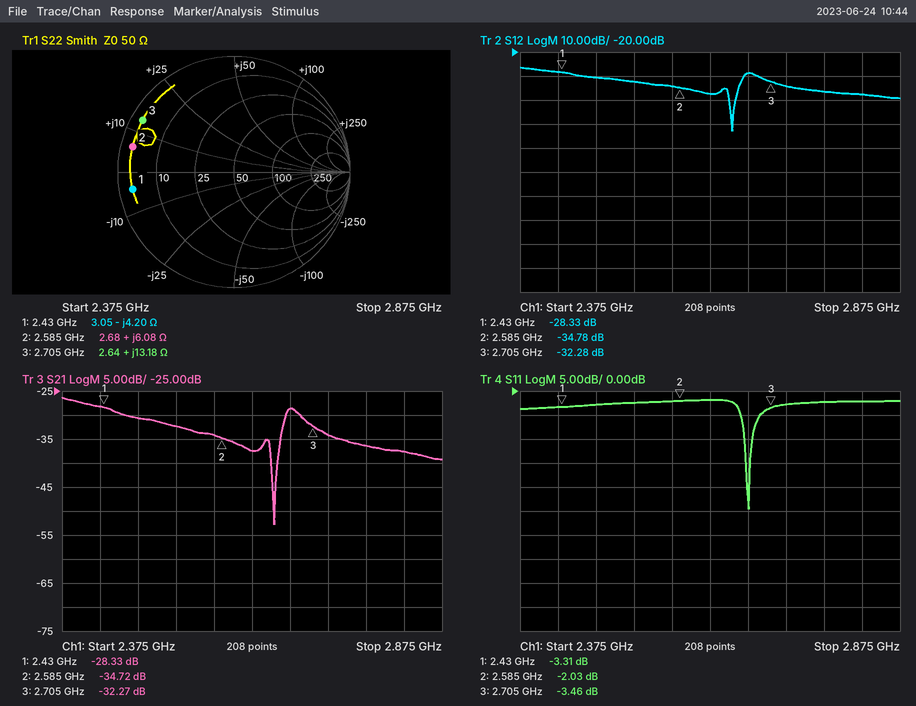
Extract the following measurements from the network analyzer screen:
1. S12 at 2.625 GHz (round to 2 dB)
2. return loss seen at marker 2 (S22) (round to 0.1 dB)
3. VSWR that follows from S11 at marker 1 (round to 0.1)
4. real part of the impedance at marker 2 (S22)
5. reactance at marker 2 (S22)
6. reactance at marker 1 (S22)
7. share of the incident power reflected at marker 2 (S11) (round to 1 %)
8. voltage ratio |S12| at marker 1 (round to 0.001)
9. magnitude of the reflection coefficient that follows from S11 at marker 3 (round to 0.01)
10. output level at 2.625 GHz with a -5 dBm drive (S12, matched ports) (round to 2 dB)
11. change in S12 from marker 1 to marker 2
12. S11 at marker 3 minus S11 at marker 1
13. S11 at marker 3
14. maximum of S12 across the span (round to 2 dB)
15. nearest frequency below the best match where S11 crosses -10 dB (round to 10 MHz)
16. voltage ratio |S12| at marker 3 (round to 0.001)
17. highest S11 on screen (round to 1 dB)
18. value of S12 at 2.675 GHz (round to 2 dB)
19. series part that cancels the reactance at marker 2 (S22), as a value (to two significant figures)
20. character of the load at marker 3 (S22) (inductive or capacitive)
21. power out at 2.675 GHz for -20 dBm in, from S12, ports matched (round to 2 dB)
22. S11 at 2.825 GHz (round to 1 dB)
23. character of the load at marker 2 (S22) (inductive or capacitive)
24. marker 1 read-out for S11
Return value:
-38 dB
0.9 dB
5.3
2.68 Ω
+6.08 Ω
-4.20 Ω
63 %
0.038
0.67
-42 dBm
-6.45 dB
-0.15 dB
-3.46 dB
-26 dB
2.67 GHz
0.024
-2 dB
-28 dB
10 pF
inductive
-48 dBm
-2 dB
inductive
-3.31 dB
